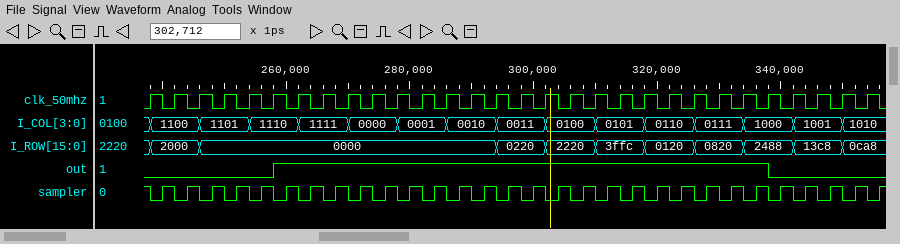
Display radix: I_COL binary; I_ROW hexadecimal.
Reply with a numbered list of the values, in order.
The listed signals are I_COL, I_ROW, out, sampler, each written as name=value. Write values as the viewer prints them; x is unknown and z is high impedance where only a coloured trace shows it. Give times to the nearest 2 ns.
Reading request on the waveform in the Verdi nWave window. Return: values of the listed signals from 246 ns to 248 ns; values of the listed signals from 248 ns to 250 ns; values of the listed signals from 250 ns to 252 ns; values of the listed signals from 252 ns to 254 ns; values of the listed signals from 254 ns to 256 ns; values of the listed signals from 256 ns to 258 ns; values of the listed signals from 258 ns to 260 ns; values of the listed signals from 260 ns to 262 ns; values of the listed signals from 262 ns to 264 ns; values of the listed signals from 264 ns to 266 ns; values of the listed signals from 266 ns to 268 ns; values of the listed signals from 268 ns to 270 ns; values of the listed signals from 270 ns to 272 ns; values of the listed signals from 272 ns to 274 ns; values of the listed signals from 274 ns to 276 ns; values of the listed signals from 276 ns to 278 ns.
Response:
1. I_COL=1101, I_ROW=0000, out=0, sampler=0
2. I_COL=1101, I_ROW=0000, out=0, sampler=1
3. I_COL=1101, I_ROW=0000, out=0, sampler=0
4. I_COL=1101, I_ROW=0000, out=0, sampler=1
5. I_COL=1110, I_ROW=0000, out=0, sampler=0
6. I_COL=1110, I_ROW=0000, out=0, sampler=1
7. I_COL=1110, I_ROW=0000, out=1, sampler=0
8. I_COL=1110, I_ROW=0000, out=1, sampler=1
9. I_COL=1111, I_ROW=0000, out=1, sampler=0
10. I_COL=1111, I_ROW=0000, out=1, sampler=1
11. I_COL=1111, I_ROW=0000, out=1, sampler=0
12. I_COL=1111, I_ROW=0000, out=1, sampler=1
13. I_COL=0000, I_ROW=0000, out=1, sampler=0
14. I_COL=0000, I_ROW=0000, out=1, sampler=1
15. I_COL=0000, I_ROW=0000, out=1, sampler=0
16. I_COL=0000, I_ROW=0000, out=1, sampler=1
